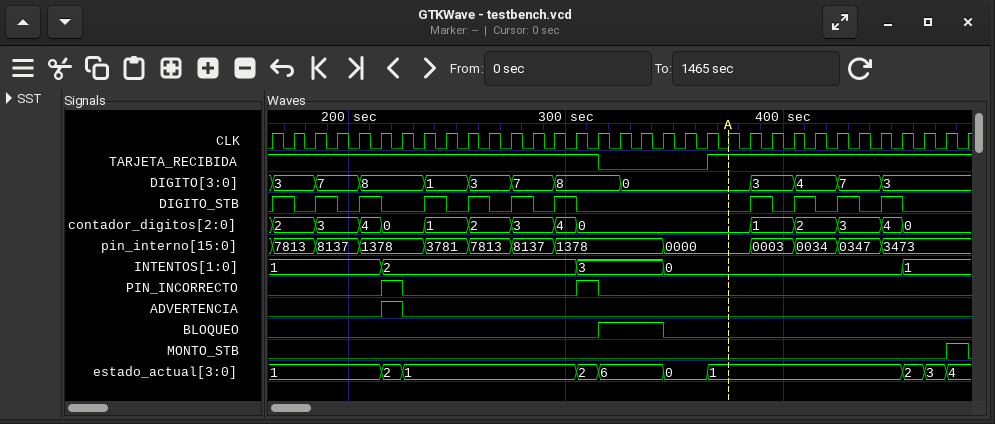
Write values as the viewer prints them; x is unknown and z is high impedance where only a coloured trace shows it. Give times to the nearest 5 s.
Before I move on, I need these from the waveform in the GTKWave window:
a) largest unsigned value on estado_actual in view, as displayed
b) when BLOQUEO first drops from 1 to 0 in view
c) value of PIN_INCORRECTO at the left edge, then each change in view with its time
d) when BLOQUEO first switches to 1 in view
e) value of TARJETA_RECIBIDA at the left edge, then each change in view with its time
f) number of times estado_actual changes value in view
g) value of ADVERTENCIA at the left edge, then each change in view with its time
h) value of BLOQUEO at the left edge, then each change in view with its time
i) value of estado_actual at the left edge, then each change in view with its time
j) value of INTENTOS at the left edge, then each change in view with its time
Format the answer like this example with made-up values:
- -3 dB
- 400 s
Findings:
- 6
- 345 s
- 0, 1 at 215 s, 0 at 225 s, 1 at 305 s, 0 at 315 s
- 315 s
- 1, 0 at 315 s, 1 at 365 s
- 9
- 0, 1 at 215 s, 0 at 225 s
- 0, 1 at 315 s, 0 at 345 s
- 1, 2 at 215 s, 1 at 225 s, 2 at 305 s, 6 at 315 s, 0 at 345 s, 1 at 365 s, 2 at 455 s, 3 at 465 s, 4 at 475 s
- 1, 2 at 215 s, 3 at 305 s, 0 at 345 s, 1 at 455 s
